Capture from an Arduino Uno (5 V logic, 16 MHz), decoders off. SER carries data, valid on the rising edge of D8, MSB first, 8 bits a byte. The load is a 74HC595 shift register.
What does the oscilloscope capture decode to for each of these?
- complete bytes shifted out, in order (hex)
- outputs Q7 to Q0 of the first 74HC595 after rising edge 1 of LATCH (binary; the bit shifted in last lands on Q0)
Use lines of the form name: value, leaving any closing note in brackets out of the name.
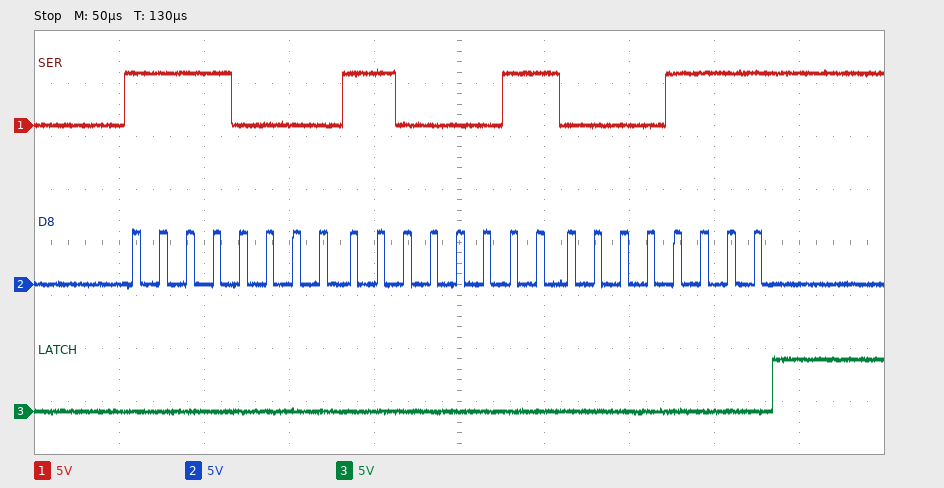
complete bytes shifted out, in order: 0xF0 0xC3 0x0F
outputs Q7 to Q0 of the first 74HC595 after rising edge 1 of LATCH: 00001111
